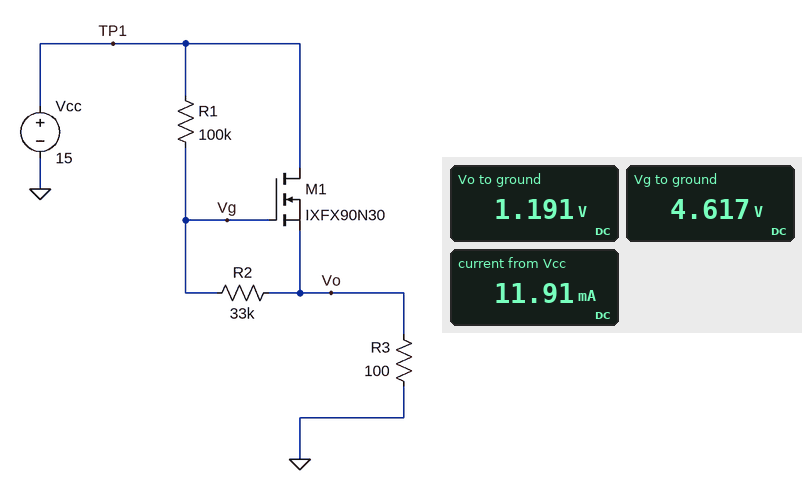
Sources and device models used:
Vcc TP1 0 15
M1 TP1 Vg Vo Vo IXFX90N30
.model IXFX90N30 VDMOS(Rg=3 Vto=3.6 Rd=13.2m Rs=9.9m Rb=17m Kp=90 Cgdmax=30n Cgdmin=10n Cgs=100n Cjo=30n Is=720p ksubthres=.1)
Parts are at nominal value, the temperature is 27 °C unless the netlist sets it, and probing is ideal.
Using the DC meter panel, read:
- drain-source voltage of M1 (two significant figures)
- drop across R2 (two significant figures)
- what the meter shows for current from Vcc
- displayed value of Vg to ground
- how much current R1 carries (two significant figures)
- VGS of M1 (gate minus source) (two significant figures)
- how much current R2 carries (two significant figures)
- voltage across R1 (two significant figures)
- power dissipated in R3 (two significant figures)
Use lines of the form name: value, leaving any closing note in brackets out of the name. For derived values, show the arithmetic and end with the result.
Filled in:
drain-source voltage of M1: 15 V - 1.191 V = 14 V
drop across R2: 4.617 V - 1.191 V = 3.4 V
what the meter shows for current from Vcc: 11.91 mA
displayed value of Vg to ground: 4.617 V
how much current R1 carries: (15 V - 4.617 V) / 100 kΩ = 100 µA
VGS of M1 (gate minus source): 4.617 V - 1.191 V = 3.4 V
how much current R2 carries: (4.617 V - 1.191 V) / 33 kΩ = 100 µA
voltage across R1: 15 V - 4.617 V = 10 V
power dissipated in R3: (1.191 V)^2 / 100 Ω = 14 mW
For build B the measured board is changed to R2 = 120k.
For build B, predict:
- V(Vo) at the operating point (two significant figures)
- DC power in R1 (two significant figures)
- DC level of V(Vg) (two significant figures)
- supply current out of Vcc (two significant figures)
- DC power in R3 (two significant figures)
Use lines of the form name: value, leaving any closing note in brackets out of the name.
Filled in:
V(Vo) at the operating point: 8.5 V
DC power in R1: 87 µW
DC level of V(Vg): 12 V
supply current out of Vcc: 85 mA
DC power in R3: 720 mW
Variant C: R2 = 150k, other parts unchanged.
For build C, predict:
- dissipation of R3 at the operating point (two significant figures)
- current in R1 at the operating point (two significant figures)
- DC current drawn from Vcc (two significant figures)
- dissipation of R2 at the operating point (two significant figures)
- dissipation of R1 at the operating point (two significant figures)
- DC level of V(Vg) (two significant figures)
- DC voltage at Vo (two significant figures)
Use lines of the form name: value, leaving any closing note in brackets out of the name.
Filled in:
dissipation of R3 at the operating point: 830 mW
current in R1 at the operating point: 24 µA
DC current drawn from Vcc: 91 mA
dissipation of R2 at the operating point: 84 µW
dissipation of R1 at the operating point: 56 µW
DC level of V(Vg): 13 V
DC voltage at Vo: 9.1 V
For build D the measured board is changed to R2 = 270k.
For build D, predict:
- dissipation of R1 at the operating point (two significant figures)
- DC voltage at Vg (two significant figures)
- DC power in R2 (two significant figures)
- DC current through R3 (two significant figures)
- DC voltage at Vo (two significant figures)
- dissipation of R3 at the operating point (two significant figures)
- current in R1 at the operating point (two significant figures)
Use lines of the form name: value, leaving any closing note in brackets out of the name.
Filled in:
dissipation of R1 at the operating point: 17 µW
DC voltage at Vg: 14 V
DC power in R2: 47 µW
DC current through R3: 100 mA
DC voltage at Vo: 10 V
dissipation of R3 at the operating point: 1.0 W
current in R1 at the operating point: 13 µA
